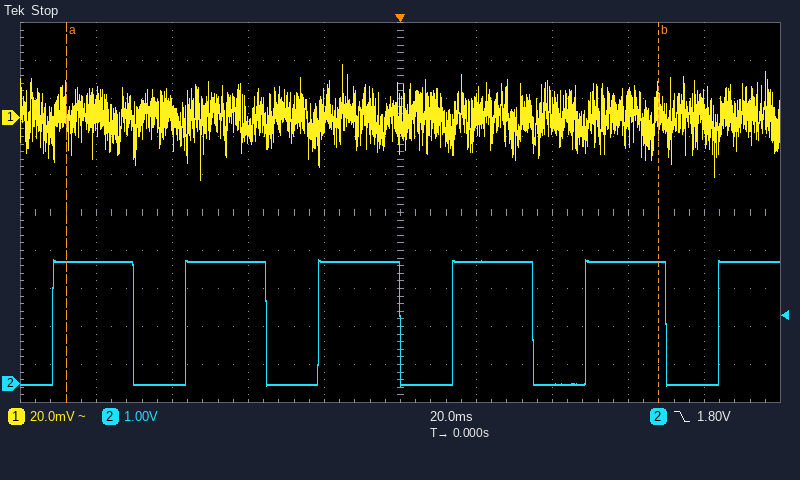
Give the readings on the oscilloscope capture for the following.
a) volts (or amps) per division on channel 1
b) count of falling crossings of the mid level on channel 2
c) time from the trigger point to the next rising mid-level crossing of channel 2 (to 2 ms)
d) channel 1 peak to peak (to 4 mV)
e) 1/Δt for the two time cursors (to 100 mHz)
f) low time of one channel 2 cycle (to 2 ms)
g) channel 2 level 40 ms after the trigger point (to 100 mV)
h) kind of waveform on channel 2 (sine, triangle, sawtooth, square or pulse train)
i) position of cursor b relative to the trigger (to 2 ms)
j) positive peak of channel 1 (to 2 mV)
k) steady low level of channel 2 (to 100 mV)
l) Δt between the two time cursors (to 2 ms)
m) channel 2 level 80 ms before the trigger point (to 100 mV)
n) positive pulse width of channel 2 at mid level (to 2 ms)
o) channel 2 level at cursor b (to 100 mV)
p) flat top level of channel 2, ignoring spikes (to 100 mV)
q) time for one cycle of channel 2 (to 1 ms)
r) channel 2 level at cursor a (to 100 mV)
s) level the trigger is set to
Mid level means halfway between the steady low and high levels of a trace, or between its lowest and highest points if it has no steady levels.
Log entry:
20 mV
5
14 ms
60 mV
6.4 Hz
14 ms
0.0 V
pulse train
+68 ms
28 mV
0.0 V
156 ms
3.2 V
22 ms
3.2 V
3.2 V
35 ms
3.2 V
1.80 V
